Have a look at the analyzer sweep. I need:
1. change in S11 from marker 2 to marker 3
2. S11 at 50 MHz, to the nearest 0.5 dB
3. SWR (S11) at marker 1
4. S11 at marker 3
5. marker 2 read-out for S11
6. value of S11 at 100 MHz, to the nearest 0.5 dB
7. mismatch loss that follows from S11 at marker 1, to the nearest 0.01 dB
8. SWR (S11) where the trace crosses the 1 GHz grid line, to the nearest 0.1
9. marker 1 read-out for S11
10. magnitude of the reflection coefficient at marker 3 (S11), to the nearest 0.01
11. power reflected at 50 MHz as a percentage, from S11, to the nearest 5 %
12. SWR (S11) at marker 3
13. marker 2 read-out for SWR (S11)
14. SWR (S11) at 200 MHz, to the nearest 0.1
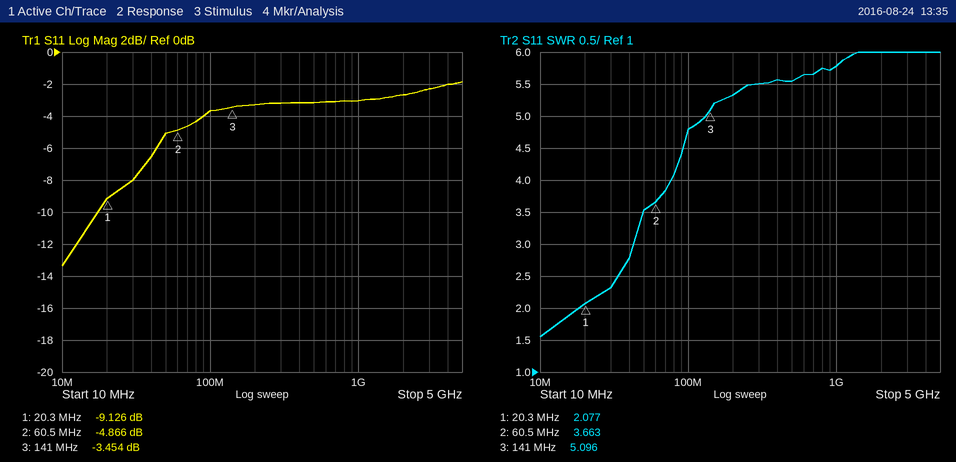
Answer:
1.412 dB
-5.0 dB
2.077
-3.454 dB
-4.866 dB
-3.5 dB
0.57 dB
5.8
-9.126 dB
0.67
30 %
5.096
3.663
5.3
